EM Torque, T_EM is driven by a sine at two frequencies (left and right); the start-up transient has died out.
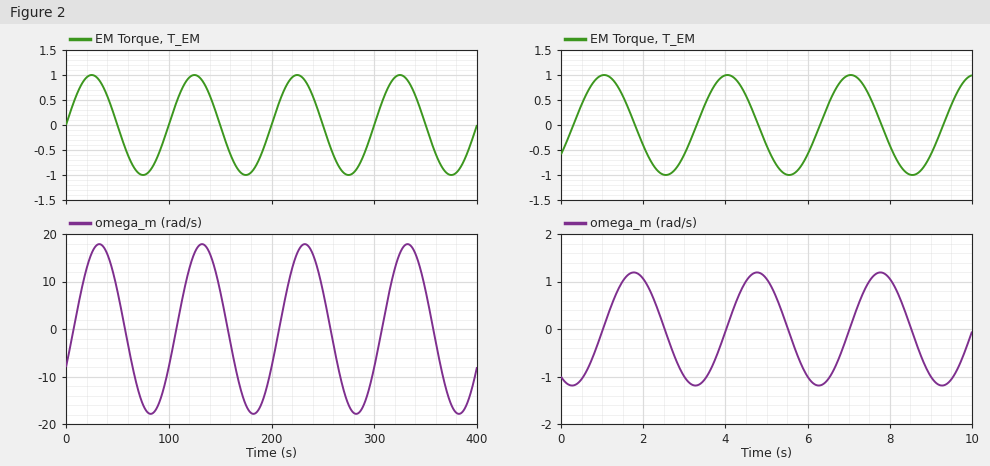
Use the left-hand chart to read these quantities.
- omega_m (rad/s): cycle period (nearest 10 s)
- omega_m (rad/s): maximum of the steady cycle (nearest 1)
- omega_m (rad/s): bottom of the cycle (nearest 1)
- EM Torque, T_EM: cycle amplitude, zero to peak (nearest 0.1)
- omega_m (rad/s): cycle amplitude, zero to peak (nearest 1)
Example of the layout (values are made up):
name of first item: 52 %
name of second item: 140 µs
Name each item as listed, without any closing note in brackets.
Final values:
omega_m (rad/s): cycle period: 100 s
omega_m (rad/s): maximum of the steady cycle: 18
omega_m (rad/s): bottom of the cycle: -18
EM Torque, T_EM: cycle amplitude, zero to peak: 1.0
omega_m (rad/s): cycle amplitude, zero to peak: 18
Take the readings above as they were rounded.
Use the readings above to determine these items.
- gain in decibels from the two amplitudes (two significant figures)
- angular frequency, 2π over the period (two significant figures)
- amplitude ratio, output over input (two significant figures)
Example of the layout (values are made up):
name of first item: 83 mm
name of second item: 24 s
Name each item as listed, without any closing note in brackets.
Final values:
gain in decibels from the two amplitudes: 25 dB
angular frequency, 2π over the period: 0.063 rad/s
amplitude ratio, output over input: 18
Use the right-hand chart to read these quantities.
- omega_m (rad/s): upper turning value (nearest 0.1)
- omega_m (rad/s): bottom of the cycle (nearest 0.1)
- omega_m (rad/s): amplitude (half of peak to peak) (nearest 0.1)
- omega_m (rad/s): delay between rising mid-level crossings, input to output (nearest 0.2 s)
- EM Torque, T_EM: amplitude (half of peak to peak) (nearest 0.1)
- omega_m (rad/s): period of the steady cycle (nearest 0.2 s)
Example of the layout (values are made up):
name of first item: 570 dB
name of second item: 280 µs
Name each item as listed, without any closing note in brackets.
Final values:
omega_m (rad/s): upper turning value: 1.2
omega_m (rad/s): bottom of the cycle: -1.2
omega_m (rad/s): amplitude (half of peak to peak): 1.2
omega_m (rad/s): delay between rising mid-level crossings, input to output: 0.8 s
EM Torque, T_EM: amplitude (half of peak to peak): 1.0
omega_m (rad/s): period of the steady cycle: 3.0 s
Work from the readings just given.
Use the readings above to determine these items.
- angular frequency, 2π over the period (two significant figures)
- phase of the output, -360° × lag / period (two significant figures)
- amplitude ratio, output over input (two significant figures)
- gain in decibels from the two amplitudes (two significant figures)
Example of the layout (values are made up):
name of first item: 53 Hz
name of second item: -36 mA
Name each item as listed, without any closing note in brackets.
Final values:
angular frequency, 2π over the period: 2.1 rad/s
phase of the output, -360° × lag / period: -96°
amplitude ratio, output over input: 1.2
gain in decibels from the two amplitudes: 1.6 dB
